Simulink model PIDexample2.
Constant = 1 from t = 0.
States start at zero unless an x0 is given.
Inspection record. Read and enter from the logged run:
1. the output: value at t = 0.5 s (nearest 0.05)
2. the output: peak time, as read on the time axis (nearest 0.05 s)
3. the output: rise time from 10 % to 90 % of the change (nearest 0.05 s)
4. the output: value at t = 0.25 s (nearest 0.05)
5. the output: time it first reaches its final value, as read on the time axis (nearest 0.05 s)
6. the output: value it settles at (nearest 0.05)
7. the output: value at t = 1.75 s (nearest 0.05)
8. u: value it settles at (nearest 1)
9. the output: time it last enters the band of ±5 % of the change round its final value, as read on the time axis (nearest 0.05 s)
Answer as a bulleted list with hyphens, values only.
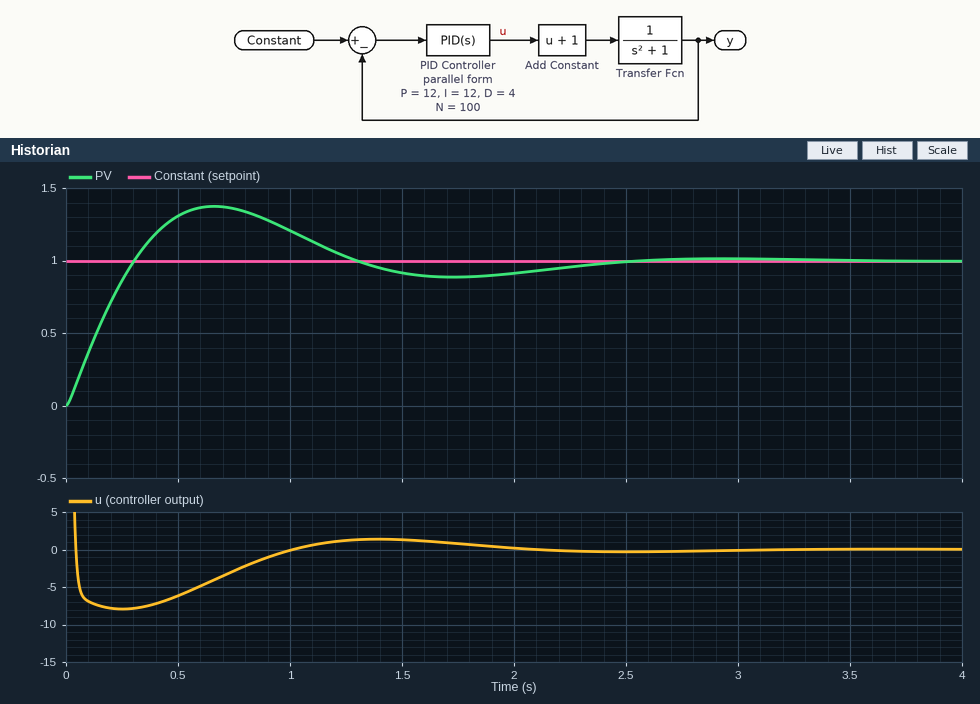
- 1.30
- 0.65 s
- 0.25 s
- 0.85
- 0.30 s
- 1.00
- 0.90
- 0
- 2.20 s
